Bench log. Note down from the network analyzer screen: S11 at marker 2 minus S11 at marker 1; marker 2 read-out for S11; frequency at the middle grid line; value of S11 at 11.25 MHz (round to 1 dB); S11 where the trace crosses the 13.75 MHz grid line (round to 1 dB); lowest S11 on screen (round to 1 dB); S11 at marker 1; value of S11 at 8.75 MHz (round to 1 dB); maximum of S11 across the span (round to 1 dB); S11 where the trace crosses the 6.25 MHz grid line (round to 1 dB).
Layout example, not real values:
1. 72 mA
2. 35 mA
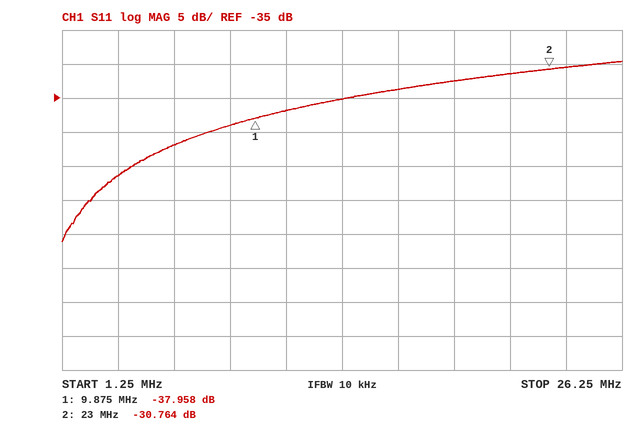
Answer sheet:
1. 7.194 dB
2. -30.764 dB
3. 13.75 MHz
4. -37 dB
5. -35 dB
6. -56 dB
7. -37.958 dB
8. -39 dB
9. -30 dB
10. -42 dB
